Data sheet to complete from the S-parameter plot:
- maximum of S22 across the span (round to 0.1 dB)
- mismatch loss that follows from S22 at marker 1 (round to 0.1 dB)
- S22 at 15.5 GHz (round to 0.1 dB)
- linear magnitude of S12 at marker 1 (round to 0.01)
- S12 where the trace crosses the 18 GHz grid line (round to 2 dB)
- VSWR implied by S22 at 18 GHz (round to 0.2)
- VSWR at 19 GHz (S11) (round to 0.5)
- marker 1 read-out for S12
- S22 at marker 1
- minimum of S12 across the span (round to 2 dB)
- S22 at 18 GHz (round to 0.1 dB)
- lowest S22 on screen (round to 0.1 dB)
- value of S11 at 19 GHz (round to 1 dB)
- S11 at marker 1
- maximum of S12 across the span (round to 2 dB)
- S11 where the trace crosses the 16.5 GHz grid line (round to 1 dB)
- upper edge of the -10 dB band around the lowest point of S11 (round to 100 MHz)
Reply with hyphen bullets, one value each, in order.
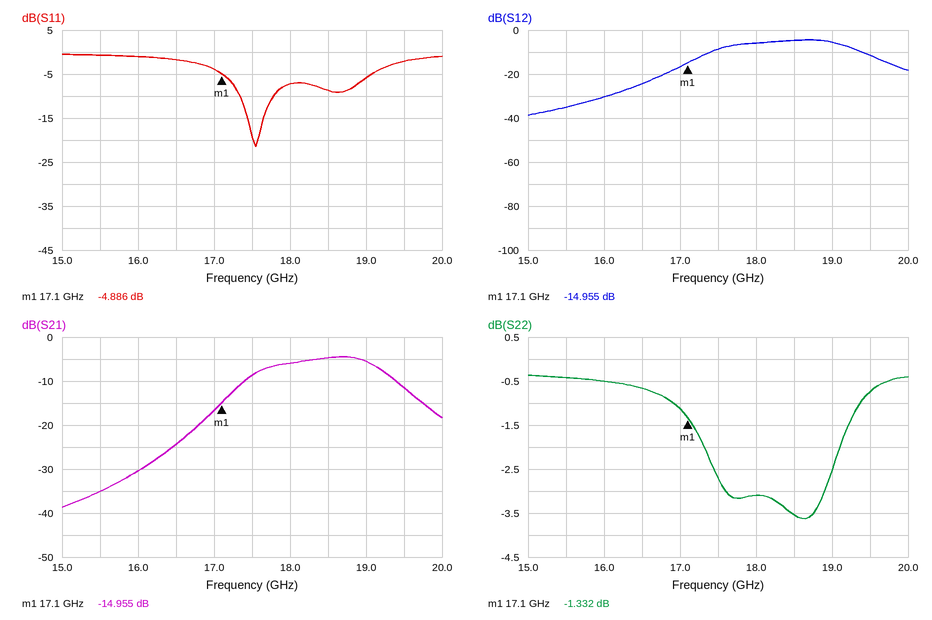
- -0.4 dB
- 5.8 dB
- -0.4 dB
- 0.18
- -6 dB
- 5.6
- 3.0
- -14.955 dB
- -1.332 dB
- -38 dB
- -3.1 dB
- -3.6 dB
- -6 dB
- -4.886 dB
- -4 dB
- -2 dB
- 17.8 GHz
